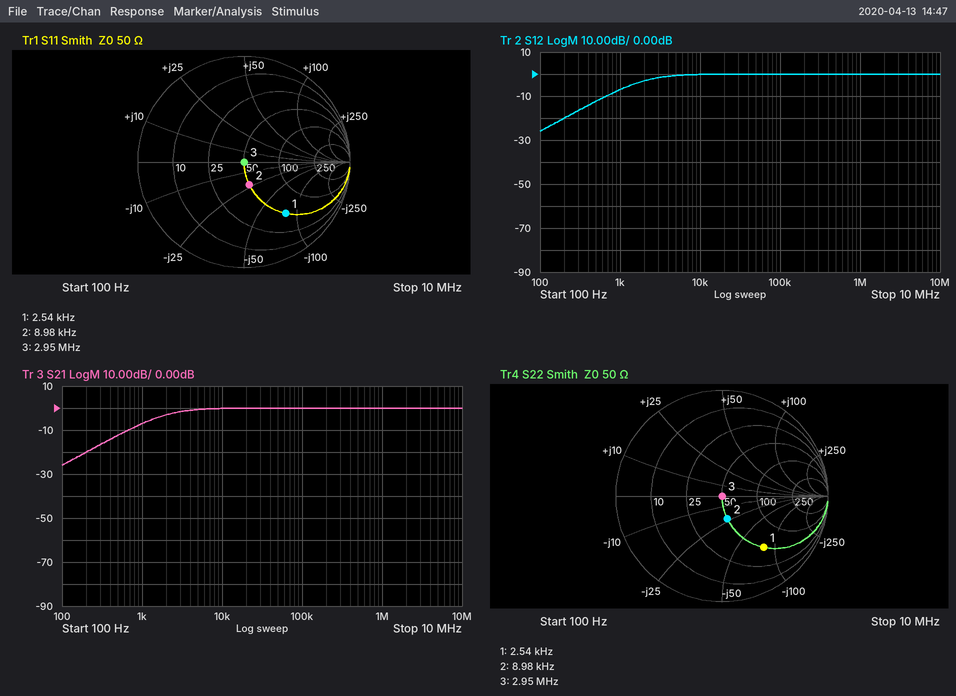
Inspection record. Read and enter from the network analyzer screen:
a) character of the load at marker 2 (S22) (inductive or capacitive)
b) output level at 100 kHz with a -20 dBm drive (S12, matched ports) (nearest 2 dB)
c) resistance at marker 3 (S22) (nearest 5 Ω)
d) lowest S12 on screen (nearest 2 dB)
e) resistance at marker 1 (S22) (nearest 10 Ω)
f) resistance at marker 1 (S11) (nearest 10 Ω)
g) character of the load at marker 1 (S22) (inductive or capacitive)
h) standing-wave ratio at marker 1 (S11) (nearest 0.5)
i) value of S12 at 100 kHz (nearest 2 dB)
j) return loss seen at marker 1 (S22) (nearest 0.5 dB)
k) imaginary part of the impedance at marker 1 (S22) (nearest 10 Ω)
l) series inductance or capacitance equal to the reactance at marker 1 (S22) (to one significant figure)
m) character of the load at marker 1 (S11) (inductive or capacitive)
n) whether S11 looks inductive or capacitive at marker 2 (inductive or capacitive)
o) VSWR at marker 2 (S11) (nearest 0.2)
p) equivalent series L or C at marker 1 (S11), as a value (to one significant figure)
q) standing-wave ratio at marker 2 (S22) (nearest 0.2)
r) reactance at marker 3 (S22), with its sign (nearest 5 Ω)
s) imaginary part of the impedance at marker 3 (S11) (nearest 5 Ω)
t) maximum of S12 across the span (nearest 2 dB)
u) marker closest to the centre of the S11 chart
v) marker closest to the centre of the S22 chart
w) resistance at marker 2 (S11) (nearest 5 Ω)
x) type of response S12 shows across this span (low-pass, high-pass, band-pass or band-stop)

capacitive
-20 dBm
50 Ω
-26 dB
50 Ω
50 Ω
capacitive
4.5
0 dB
4.0 dB
-80 Ω
800 nF
capacitive
capacitive
1.6
800 nF
1.6
0 Ω
0 Ω
0 dB
marker 3
marker 3
50 Ω
high-pass
